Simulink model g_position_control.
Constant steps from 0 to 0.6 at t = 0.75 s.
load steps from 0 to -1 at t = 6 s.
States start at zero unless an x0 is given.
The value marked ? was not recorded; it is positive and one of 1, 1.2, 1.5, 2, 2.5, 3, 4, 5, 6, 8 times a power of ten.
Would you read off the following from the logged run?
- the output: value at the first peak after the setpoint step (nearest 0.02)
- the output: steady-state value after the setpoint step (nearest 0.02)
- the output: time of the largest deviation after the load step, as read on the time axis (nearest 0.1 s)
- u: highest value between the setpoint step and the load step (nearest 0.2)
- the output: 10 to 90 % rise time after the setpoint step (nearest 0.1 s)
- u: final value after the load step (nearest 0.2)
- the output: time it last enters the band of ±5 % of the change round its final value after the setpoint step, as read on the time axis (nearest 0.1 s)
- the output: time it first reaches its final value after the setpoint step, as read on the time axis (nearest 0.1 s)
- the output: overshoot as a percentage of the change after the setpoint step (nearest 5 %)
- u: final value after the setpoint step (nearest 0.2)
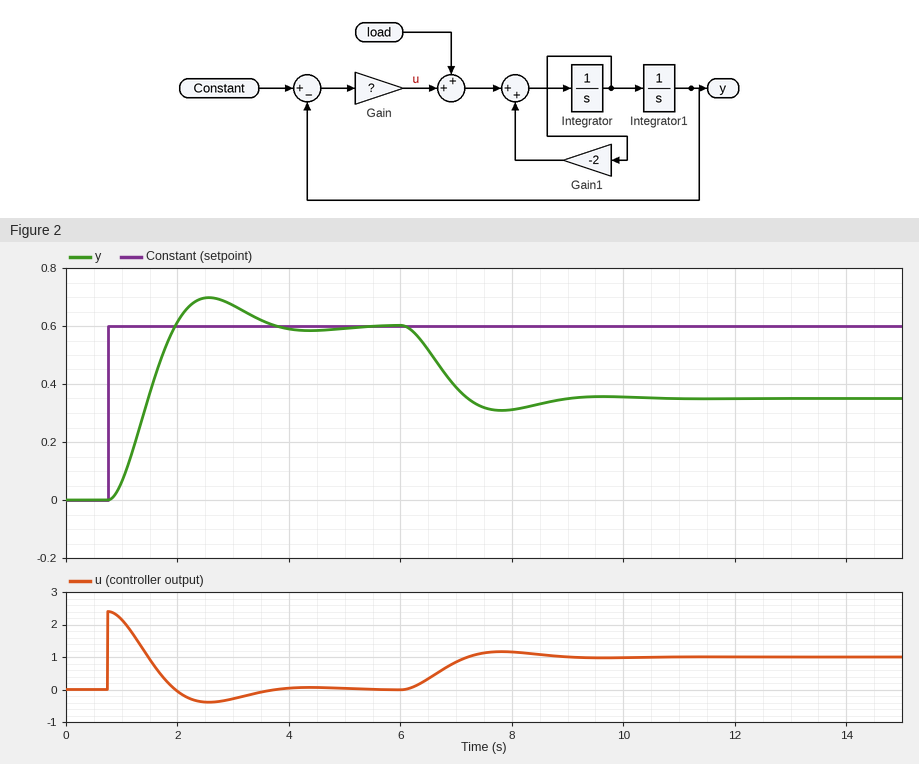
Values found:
0.70
0.60
7.8 s
2.4
0.8 s
1.0
3.4 s
2.0 s
15 %
0.0
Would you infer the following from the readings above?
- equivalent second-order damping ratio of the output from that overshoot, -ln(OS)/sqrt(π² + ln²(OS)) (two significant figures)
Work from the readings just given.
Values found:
0.52
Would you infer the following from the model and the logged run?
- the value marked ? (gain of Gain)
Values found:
4
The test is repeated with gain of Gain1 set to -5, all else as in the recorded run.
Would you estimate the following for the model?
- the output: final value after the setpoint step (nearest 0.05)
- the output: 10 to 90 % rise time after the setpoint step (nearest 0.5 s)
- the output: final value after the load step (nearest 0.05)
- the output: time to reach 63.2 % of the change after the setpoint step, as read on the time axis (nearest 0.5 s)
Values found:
0.60
2.5 s
0.35
2.0 s
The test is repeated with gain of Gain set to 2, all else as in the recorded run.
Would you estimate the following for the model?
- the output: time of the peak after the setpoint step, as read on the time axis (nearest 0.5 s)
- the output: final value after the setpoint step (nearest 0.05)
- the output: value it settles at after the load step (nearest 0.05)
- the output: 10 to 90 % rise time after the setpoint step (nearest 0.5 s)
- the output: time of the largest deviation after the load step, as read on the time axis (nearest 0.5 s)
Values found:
4.0 s
0.60
0.10
1.5 s
9.0 s
